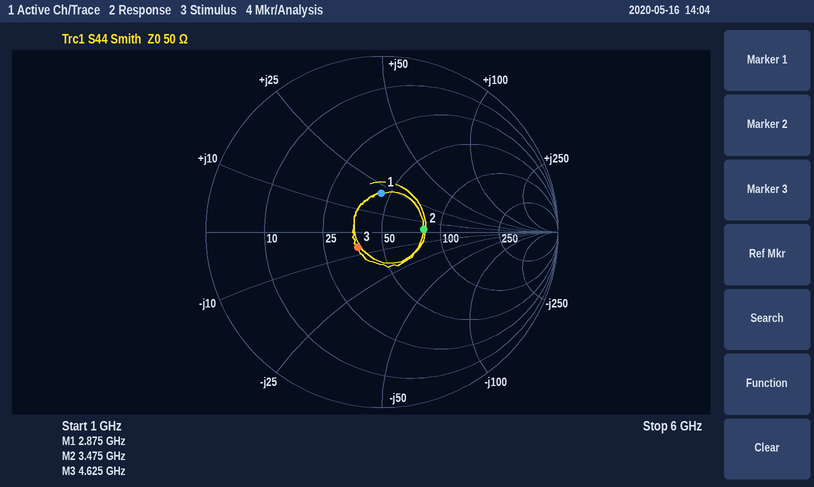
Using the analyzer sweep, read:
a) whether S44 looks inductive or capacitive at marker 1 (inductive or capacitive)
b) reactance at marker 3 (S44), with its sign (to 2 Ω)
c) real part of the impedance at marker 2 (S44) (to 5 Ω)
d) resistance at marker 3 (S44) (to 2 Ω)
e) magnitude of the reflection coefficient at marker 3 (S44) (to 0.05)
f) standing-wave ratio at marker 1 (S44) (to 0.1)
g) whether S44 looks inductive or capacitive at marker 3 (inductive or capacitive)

inductive
-6 Ω
80 Ω
38 Ω
0.15
1.6
capacitive
